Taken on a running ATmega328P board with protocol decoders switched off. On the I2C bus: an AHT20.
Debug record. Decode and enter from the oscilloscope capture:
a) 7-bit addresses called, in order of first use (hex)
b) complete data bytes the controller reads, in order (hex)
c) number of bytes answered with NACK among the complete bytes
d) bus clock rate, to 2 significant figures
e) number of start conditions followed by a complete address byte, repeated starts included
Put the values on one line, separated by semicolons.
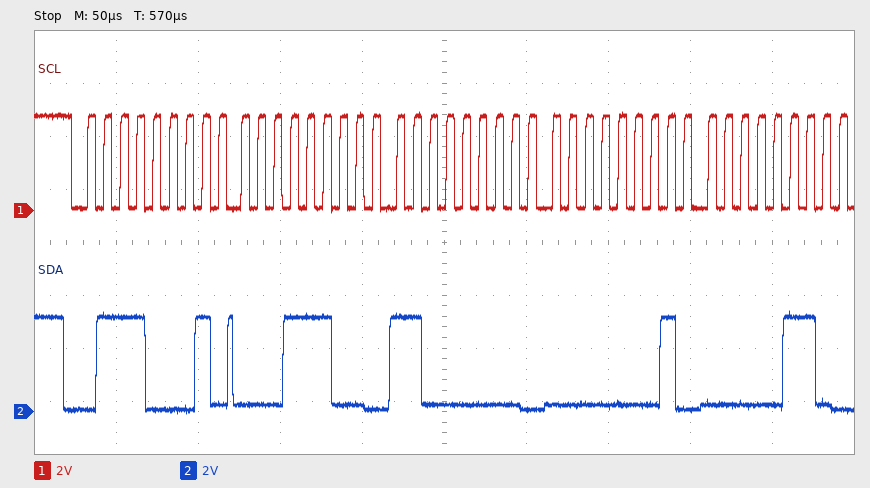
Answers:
0x38; 1C C0 01 06; 0; 100 kHz; 1
